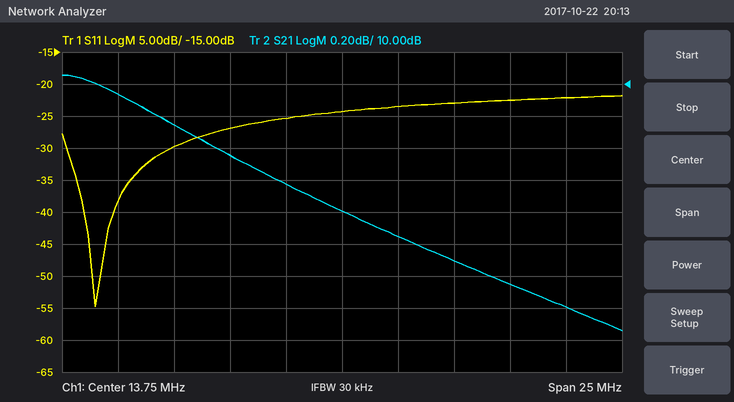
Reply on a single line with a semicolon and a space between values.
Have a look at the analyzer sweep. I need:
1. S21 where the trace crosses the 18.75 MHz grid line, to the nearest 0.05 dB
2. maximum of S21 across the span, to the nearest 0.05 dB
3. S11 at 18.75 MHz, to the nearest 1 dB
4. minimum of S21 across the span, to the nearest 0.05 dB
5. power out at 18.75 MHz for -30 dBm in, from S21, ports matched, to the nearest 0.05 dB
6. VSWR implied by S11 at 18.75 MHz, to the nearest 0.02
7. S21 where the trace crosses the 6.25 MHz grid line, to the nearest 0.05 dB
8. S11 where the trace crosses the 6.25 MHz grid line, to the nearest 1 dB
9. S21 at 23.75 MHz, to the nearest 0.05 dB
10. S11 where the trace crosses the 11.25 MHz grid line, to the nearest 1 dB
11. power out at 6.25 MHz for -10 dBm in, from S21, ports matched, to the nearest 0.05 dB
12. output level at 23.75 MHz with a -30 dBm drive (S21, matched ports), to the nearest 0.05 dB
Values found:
8.90 dB; 10.05 dB; -23 dB; 8.45 dB; -21.10 dBm; 1.16; 9.75 dB; -30 dB; 8.60 dB; -25 dB; -0.25 dBm; -21.40 dBm
